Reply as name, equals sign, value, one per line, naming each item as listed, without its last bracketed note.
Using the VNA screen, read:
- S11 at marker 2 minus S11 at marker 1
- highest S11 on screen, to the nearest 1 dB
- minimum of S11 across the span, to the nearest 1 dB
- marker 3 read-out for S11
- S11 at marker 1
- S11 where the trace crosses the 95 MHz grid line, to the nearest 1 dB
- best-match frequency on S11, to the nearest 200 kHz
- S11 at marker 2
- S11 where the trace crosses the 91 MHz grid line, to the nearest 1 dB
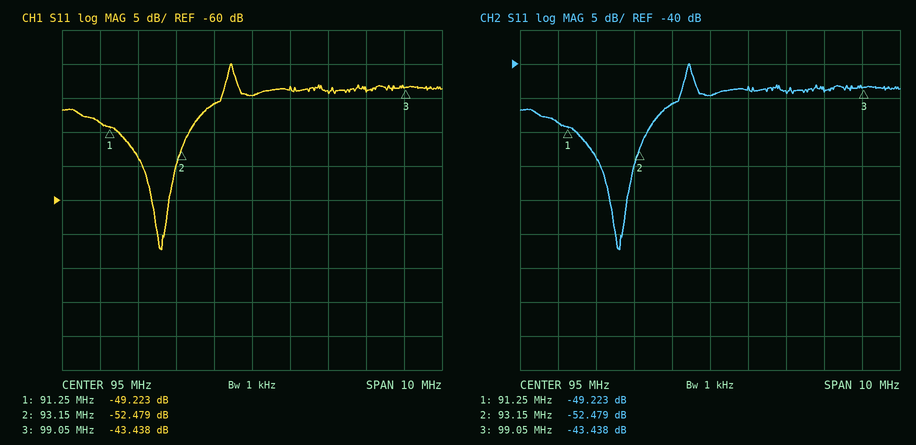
S11 at marker 2 minus S11 at marker 1 = -3.256 dB
highest S11 on screen, to the nearest 1 dB = -40 dB
minimum of S11 across the span, to the nearest 1 dB = -67 dB
marker 3 read-out for S11 = -43.438 dB
S11 at marker 1 = -49.223 dB
S11 where the trace crosses the 95 MHz grid line, to the nearest 1 dB = -45 dB
best-match frequency on S11, to the nearest 200 kHz = 92.6 MHz
S11 at marker 2 = -52.479 dB
S11 where the trace crosses the 91 MHz grid line, to the nearest 1 dB = -49 dB
